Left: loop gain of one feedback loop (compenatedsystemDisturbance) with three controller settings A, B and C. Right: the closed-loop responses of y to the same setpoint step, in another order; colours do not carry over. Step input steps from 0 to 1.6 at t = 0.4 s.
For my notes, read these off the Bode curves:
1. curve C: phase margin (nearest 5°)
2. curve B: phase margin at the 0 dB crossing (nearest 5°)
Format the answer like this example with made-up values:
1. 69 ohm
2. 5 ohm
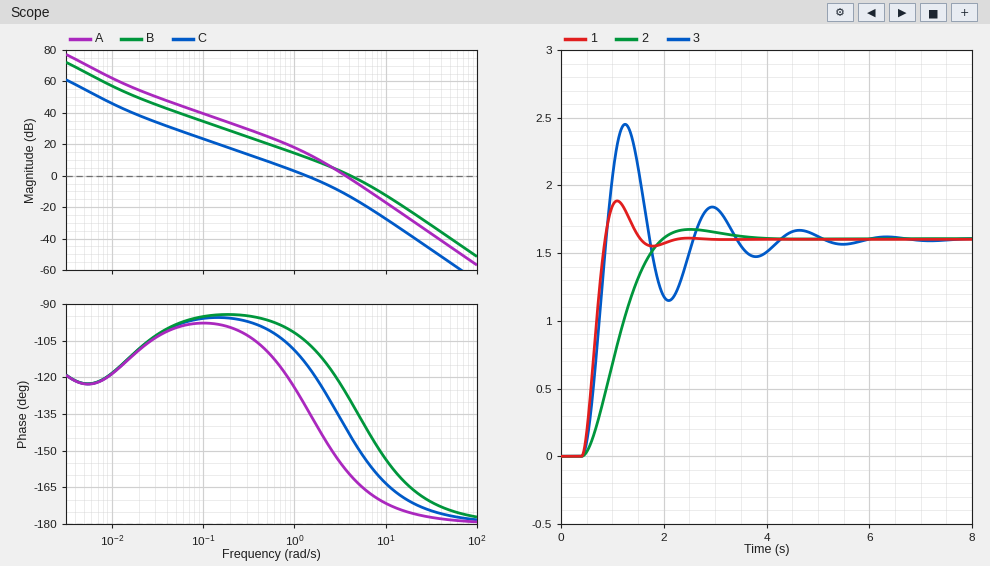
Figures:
1. 65°
2. 50°
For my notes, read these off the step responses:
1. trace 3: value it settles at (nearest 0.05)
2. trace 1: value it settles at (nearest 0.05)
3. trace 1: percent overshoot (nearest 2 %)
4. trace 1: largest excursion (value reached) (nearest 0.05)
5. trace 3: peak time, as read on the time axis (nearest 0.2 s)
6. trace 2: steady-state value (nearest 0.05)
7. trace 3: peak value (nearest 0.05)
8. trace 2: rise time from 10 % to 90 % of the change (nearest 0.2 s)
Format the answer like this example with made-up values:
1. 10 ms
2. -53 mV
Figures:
1. 1.60
2. 1.60
3. 18 %
4. 1.90
5. 1.2 s
6. 1.60
7. 2.45
8. 1.0 s
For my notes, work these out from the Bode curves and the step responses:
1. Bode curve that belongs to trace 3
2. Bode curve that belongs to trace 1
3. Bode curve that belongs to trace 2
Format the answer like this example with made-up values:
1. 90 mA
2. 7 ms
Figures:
1. A
2. B
3. C
